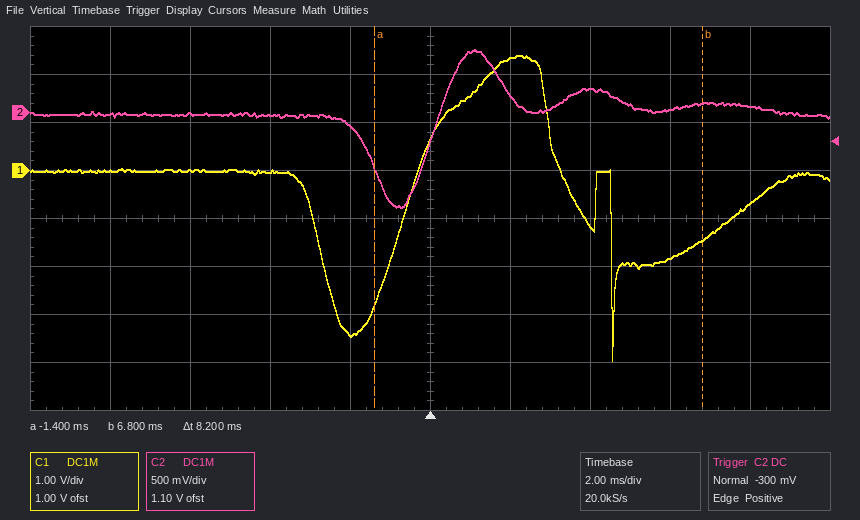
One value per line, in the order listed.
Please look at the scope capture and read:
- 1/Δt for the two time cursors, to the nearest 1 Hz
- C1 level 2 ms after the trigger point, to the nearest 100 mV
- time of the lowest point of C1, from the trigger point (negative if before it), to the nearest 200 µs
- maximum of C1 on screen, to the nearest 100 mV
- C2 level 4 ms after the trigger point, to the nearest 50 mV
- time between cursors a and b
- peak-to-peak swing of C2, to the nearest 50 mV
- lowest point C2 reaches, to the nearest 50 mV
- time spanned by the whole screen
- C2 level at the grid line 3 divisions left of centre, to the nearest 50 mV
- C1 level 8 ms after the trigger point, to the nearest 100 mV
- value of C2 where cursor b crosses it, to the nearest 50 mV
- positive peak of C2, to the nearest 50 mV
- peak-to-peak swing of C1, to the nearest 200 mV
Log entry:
122 Hz
2.3 V
+4.6 ms
2.4 V
250 mV
8.2 ms
1.65 V
-1.00 V
20 ms
0 mV
-700 mV
100 mV
650 mV
6.4 V
